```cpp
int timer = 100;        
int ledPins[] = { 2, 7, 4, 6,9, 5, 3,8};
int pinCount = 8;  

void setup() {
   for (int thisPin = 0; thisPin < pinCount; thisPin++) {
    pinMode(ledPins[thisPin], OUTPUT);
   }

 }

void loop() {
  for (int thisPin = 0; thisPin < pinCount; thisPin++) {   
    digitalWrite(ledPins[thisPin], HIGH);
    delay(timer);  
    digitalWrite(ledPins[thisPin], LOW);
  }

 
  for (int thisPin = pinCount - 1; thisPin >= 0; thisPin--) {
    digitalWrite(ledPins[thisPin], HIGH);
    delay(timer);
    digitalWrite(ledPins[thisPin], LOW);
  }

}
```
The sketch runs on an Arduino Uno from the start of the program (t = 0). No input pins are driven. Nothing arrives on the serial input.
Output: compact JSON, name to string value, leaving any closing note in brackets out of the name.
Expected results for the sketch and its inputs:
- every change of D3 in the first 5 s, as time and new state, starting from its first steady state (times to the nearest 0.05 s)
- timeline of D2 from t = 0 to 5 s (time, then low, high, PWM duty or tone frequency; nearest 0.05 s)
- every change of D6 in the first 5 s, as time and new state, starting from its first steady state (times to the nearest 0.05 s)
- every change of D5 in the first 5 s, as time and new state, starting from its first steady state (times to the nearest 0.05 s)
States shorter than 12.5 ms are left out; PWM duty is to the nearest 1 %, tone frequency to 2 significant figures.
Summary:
{"every change of D3 in the first 5 s, as time and new state, starting from its first steady state": "0 s low; 0.6 s high; 0.7 s low; 0.9 s high; 1 s low; 2.2 s high; 2.3 s low; 2.5 s high; 2.6 s low; 3.8 s high; 3.9 s low; 4.1 s high; 4.2 s low", "timeline of D2 from t = 0 to 5 s": "0 s high; 0.1 s low; 1.5 s high; 1.7 s low; 3.1 s high; 3.3 s low; 4.7 s high; 4.9 s low", "every change of D6 in the first 5 s, as time and new state, starting from its first steady state": "0 s low; 0.3 s high; 0.4 s low; 1.2 s high; 1.3 s low; 1.9 s high; 2 s low; 2.8 s high; 2.9 s low; 3.5 s high; 3.6 s low; 4.4 s high; 4.5 s low", "every change of D5 in the first 5 s, as time and new state, starting from its first steady state": "0 s low; 0.5 s high; 0.6 s low; 1 s high; 1.1 s low; 2.1 s high; 2.2 s low; 2.6 s high; 2.7 s low; 3.7 s high; 3.8 s low; 4.2 s high; 4.3 s low"}
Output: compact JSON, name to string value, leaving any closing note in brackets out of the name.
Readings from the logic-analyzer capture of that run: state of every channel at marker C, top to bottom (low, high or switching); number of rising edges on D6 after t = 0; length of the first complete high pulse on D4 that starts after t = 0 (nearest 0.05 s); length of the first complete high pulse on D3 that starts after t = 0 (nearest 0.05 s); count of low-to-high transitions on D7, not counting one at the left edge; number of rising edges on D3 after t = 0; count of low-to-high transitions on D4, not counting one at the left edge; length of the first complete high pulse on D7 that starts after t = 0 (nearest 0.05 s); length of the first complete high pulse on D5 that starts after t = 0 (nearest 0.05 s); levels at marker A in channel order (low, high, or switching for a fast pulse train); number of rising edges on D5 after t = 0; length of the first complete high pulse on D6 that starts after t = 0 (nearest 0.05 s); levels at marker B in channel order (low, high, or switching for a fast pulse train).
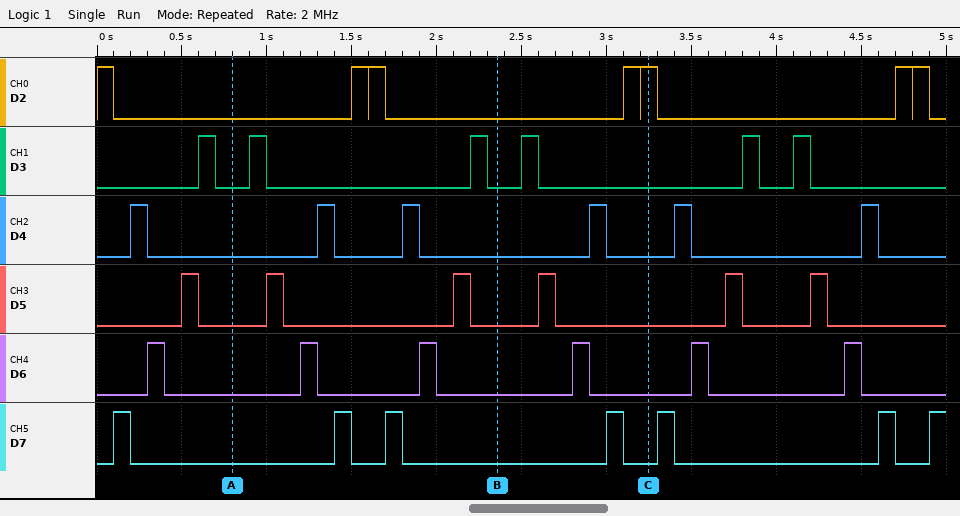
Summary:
{"state of every channel at marker C, top to bottom": "D2 high, D3 low, D4 low, D5 low, D6 low, D7 low", "number of rising edges on D6 after t = 0": "6", "length of the first complete high pulse on D4 that starts after t = 0": "0.10 s", "length of the first complete high pulse on D3 that starts after t = 0": "0.10 s", "count of low-to-high transitions on D7, not counting one at the left edge": "7", "number of rising edges on D3 after t = 0": "6", "count of low-to-high transitions on D4, not counting one at the left edge": "6", "length of the first complete high pulse on D7 that starts after t = 0": "0.10 s", "length of the first complete high pulse on D5 that starts after t = 0": "0.10 s", "levels at marker A in channel order": "D2 low, D3 low, D4 low, D5 low, D6 low, D7 low", "number of rising edges on D5 after t = 0": "6", "length of the first complete high pulse on D6 that starts after t = 0": "0.10 s", "levels at marker B in channel order": "D2 low, D3 low, D4 low, D5 low, D6 low, D7 low"}
